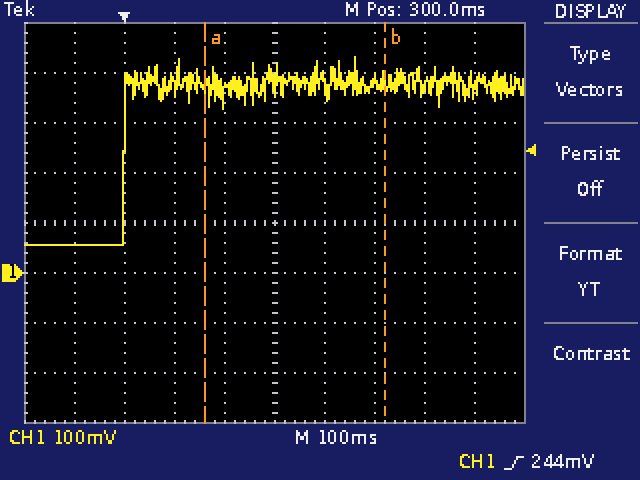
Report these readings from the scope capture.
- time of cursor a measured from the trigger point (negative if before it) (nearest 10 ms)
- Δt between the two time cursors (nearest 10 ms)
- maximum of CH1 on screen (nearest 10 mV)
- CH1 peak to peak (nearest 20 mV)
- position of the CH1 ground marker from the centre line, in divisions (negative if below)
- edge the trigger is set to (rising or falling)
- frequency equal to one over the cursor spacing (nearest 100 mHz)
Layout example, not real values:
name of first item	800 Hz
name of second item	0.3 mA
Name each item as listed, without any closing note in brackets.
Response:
time of cursor a measured from the trigger point (negative if before it)	+160 ms
Δt between the two time cursors	360 ms
maximum of CH1 on screen	430 mV
CH1 peak to peak	380 mV
position of the CH1 ground marker from the centre line, in divisions	-1.0 div
edge the trigger is set to	rising
frequency equal to one over the cursor spacing	2.8 Hz
